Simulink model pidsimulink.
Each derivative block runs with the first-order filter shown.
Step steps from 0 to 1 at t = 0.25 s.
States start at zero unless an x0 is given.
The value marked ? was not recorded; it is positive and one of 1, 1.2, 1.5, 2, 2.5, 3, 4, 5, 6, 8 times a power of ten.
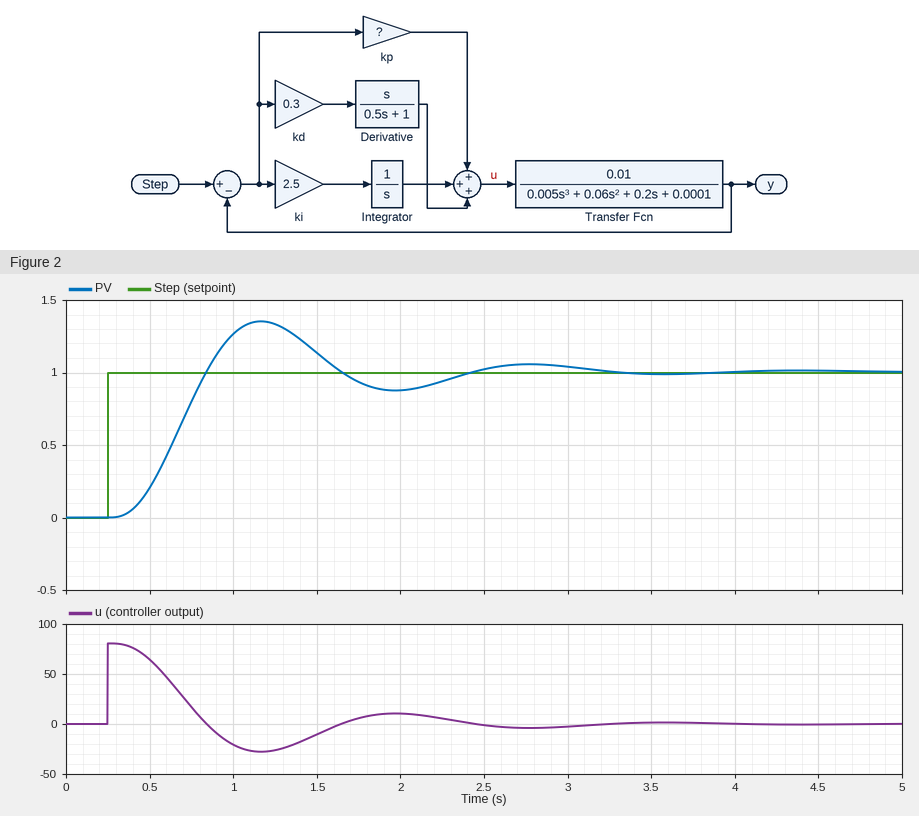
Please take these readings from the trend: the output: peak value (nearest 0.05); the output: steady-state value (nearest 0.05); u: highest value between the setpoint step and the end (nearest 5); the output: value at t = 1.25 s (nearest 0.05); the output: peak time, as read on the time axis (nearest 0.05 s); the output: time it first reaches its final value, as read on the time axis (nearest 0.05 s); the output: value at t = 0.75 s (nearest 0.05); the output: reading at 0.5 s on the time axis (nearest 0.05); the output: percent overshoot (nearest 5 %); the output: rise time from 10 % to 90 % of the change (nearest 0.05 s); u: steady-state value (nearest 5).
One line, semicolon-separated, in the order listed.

1.35; 1.00; 80; 1.35; 1.15 s; 0.85 s; 0.80; 0.20; 35 %; 0.35 s; 0
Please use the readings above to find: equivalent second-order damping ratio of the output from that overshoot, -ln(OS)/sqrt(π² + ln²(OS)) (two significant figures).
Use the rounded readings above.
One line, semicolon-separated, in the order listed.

0.32
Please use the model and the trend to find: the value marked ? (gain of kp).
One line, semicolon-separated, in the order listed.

80
